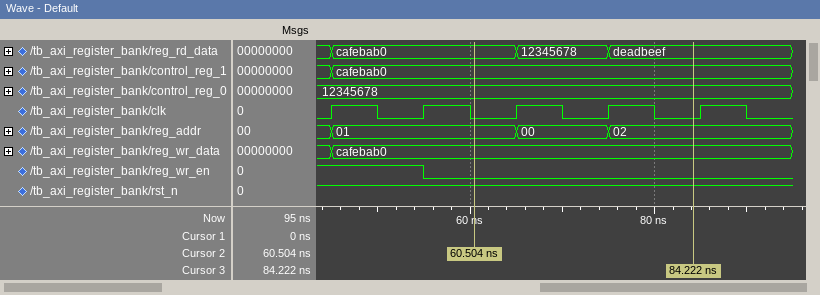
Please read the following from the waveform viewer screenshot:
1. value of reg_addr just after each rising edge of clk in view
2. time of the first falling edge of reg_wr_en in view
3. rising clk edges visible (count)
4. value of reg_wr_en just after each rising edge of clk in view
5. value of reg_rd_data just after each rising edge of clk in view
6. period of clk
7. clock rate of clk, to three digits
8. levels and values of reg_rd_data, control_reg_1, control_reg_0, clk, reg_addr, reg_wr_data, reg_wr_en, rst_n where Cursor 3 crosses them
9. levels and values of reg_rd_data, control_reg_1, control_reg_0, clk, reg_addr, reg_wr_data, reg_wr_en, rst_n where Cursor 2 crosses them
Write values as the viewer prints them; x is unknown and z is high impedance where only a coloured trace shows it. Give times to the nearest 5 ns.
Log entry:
01, 01, 00, 02, 02
55 ns
5
1 0 0 0 0
cafebab0, cafebab0, 12345678, deadbeef, deadbeef
10 ns
100 MHz
reg_rd_data=deadbeef, control_reg_1=cafebab0, control_reg_0=12345678, clk=0, reg_addr=02, reg_wr_data=cafebab0, reg_wr_en=0, rst_n=1
reg_rd_data=cafebab0, control_reg_1=cafebab0, control_reg_0=12345678, clk=0, reg_addr=01, reg_wr_data=cafebab0, reg_wr_en=0, rst_n=1
